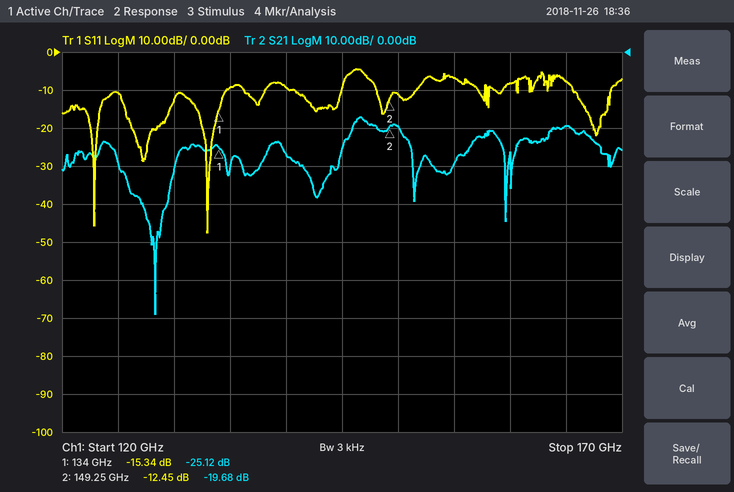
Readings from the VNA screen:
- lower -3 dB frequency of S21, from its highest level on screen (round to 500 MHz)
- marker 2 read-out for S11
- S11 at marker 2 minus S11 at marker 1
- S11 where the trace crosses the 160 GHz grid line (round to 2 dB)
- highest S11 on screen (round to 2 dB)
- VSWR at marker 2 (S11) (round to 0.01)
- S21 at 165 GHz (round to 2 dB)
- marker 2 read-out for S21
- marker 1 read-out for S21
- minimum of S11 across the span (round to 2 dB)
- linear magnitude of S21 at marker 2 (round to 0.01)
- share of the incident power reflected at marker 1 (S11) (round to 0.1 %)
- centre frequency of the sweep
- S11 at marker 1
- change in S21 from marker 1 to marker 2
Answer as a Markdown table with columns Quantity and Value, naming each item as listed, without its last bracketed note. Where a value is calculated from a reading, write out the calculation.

| Quantity | Value |
|---|---|
| lower -3 dB frequency of S21, from its highest level on screen | 146.0 GHz |
| marker 2 read-out for S11 | -12.45 dB |
| S11 at marker 2 minus S11 at marker 1 | -12.45 − (-15.34) = 2.89 dB |
| S11 where the trace crosses the 160 GHz grid line | -8 dB |
| highest S11 on screen | -4 dB |
| VSWR at marker 2 (S11) | (1 + 0.2385)/(1 − 0.2385) ≈ 1.63 |
| S21 at 165 GHz | -20 dB |
| marker 2 read-out for S21 | -19.68 dB |
| marker 1 read-out for S21 | -25.12 dB |
| minimum of S11 across the span | -48 dB |
| linear magnitude of S21 at marker 2 | 10^(-19.68/20) ≈ 0.10 |
| share of the incident power reflected at marker 1 (S11) | 10^(-15.34/10) ≈ 2.9 % |
| centre frequency of the sweep | 145 GHz |
| S11 at marker 1 | -15.34 dB |
| change in S21 from marker 1 to marker 2 | -19.68 − (-25.12) = 5.44 dB |
